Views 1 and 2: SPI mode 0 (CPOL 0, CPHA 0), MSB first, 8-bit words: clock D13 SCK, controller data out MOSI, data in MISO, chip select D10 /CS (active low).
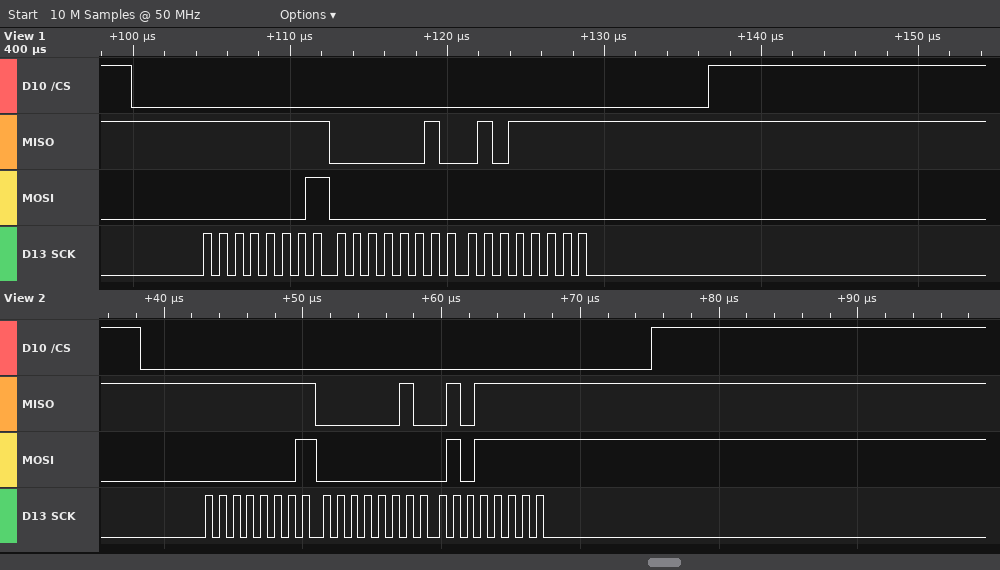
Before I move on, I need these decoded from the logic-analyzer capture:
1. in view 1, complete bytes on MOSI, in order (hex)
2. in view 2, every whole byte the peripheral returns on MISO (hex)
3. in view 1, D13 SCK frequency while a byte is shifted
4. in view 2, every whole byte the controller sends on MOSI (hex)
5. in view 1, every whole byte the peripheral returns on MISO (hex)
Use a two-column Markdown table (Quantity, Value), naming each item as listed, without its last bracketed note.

| Quantity | Value |
|---|---|
| in view 1, complete bytes on MOSI, in order | 01 00 00 |
| in view 2, every whole byte the peripheral returns on MISO | FF 02 5F |
| in view 1, D13 SCK frequency while a byte is shifted | 1 MHz |
| in view 2, every whole byte the controller sends on MOSI | 01 00 5F |
| in view 1, every whole byte the peripheral returns on MISO | FF 02 5F |
